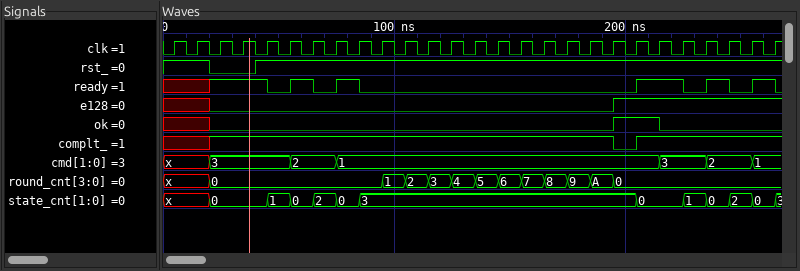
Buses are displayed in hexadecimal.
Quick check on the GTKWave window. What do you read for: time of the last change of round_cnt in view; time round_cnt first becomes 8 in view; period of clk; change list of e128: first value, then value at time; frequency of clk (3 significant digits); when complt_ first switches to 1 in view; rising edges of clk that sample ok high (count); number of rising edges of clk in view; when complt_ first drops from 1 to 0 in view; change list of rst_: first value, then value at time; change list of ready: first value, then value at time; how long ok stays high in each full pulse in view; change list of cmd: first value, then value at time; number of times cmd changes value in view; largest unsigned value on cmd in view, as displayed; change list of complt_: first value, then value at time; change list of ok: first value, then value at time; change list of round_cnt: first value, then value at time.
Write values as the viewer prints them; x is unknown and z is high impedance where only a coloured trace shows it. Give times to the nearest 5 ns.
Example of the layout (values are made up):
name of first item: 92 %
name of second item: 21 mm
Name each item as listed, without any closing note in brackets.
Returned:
time of the last change of round_cnt in view: 195 ns
time round_cnt first becomes 8 in view: 165 ns
period of clk: 10 ns
change list of e128: first value, then value at time: x, 0 at 20 ns, 1 at 195 ns
frequency of clk: 100 MHz
when complt_ first switches to 1 in view: 20 ns
rising edges of clk that sample ok high: 2
number of rising edges of clk in view: 27
when complt_ first drops from 1 to 0 in view: 195 ns
change list of rst_: first value, then value at time: 1, 0 at 20 ns, 1 at 40 ns
change list of ready: first value, then value at time: x, 1 at 20 ns, 0 at 45 ns, 1 at 55 ns, 0 at 65 ns, 1 at 75 ns, 0 at 85 ns, 1 at 205 ns, 0 at 225 ns, 1 at 235 ns, 0 at 245 ns, 1 at 255 ns, 0 at 265 ns
how long ok stays high in each full pulse in view: 20 ns
change list of cmd: first value, then value at time: x, 3 at 20 ns, 2 at 55 ns, 1 at 75 ns, 3 at 215 ns, 2 at 235 ns, 1 at 255 ns
number of times cmd changes value in view: 6
largest unsigned value on cmd in view, as displayed: 3
change list of complt_: first value, then value at time: x, 1 at 20 ns, 0 at 195 ns, 1 at 205 ns
change list of ok: first value, then value at time: x, 0 at 20 ns, 1 at 195 ns, 0 at 215 ns
change list of round_cnt: first value, then value at time: x, 0 at 20 ns, 1 at 95 ns, 2 at 105 ns, 3 at 115 ns, 4 at 125 ns, 5 at 135 ns, 6 at 145 ns, 7 at 155 ns, 8 at 165 ns, 9 at 175 ns, A at 185 ns, 0 at 195 ns
